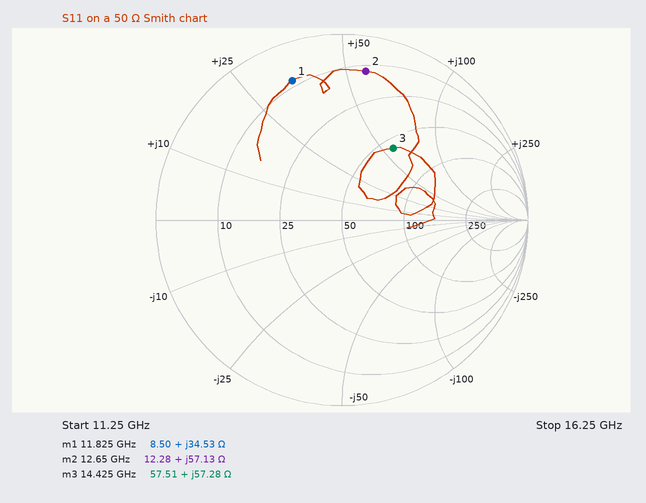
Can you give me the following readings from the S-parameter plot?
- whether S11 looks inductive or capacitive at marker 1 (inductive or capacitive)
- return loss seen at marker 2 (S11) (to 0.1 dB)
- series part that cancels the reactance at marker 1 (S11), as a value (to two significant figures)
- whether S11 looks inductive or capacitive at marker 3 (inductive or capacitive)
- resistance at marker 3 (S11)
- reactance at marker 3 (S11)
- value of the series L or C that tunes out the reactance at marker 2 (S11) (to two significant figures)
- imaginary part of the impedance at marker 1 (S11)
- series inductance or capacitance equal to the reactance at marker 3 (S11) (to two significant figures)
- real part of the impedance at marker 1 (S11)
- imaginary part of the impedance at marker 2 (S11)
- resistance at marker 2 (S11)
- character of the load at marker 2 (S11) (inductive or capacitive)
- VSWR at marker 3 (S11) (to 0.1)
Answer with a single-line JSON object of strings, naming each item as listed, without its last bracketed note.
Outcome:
{"whether S11 looks inductive or capacitive at marker 1": "inductive", "return loss seen at marker 2 (S11)": "1.8 dB", "series part that cancels the reactance at marker 1 (S11), as a value": "390 fF", "whether S11 looks inductive or capacitive at marker 3": "inductive", "resistance at marker 3": "57.51 Ω", "reactance at marker 3": "+57.28 Ω", "value of the series L or C that tunes out the reactance at marker 2 (S11)": "220 fF", "imaginary part of the impedance at marker 1": "+34.53 Ω", "series inductance or capacitance equal to the reactance at marker 3 (S11)": "630 pH", "real part of the impedance at marker 1": "8.50 Ω", "imaginary part of the impedance at marker 2": "+57.13 Ω", "resistance at marker 2": "12.28 Ω", "character of the load at marker 2 (S11)": "inductive", "VSWR at marker 3 (S11)": "2.8"}
